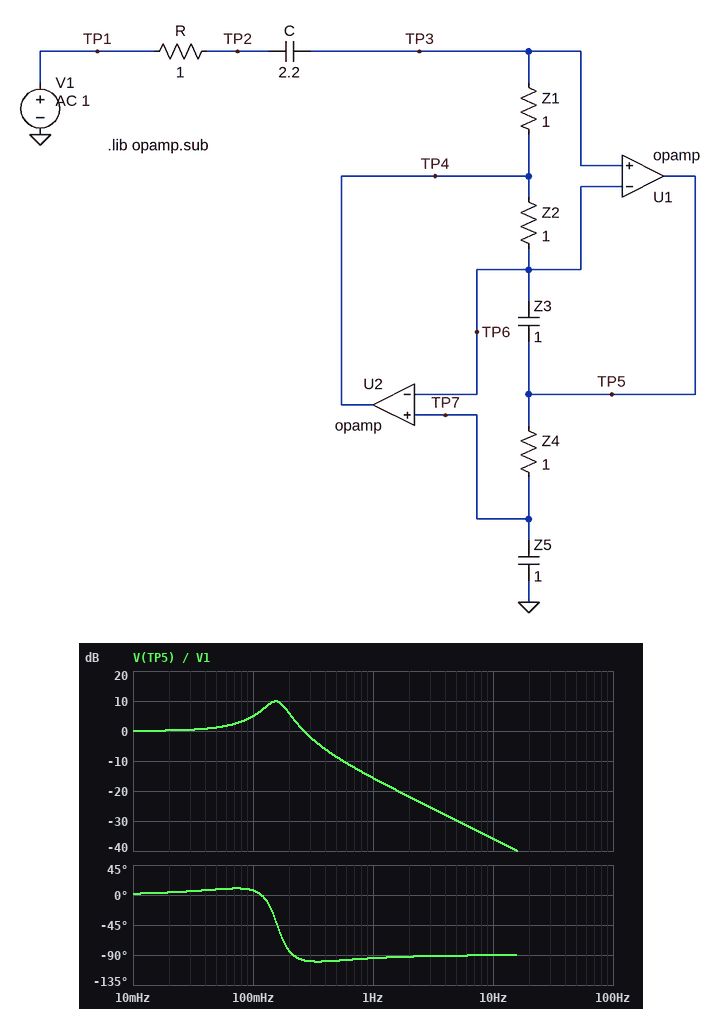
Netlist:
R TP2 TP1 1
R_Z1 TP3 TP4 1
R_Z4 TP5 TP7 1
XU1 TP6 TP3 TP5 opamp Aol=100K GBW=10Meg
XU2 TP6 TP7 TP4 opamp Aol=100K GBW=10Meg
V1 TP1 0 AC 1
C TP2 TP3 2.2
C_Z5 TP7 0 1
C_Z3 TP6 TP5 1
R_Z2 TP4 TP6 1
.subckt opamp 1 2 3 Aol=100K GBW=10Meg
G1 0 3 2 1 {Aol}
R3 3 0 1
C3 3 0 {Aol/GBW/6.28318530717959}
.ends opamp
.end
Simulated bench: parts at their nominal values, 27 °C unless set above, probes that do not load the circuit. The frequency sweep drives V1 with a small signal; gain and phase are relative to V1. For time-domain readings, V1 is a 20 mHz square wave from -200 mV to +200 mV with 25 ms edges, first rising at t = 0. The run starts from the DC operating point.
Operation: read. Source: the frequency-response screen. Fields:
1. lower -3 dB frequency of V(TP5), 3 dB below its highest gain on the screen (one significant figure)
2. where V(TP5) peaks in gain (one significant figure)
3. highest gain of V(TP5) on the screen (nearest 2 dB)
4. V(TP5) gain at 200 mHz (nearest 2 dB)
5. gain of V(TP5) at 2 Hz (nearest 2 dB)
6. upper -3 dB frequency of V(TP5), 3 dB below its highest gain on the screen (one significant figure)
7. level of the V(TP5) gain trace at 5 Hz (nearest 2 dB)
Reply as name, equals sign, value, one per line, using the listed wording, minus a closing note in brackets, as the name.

lower -3 dB frequency of V(TP5), 3 dB below its highest gain on the screen = 100 mHz
where V(TP5) peaks in gain = 200 mHz
highest gain of V(TP5) on the screen = 10 dB
V(TP5) gain at 200 mHz = 6 dB
gain of V(TP5) at 2 Hz = -22 dB
upper -3 dB frequency of V(TP5), 3 dB below its highest gain on the screen = 200 mHz
level of the V(TP5) gain trace at 5 Hz = -30 dB
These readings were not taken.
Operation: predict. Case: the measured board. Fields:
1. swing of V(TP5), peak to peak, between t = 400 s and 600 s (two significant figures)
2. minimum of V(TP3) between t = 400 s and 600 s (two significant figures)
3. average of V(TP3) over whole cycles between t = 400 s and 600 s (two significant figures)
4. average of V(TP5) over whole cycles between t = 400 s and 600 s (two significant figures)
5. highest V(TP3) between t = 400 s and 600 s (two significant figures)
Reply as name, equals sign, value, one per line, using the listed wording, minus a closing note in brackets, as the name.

swing of V(TP5), peak to peak, between t = 400 s and 600 s = 990 mV
minimum of V(TP3) between t = 400 s and 600 s = -190 mV
average of V(TP3) over whole cycles between t = 400 s and 600 s = 200 mV
average of V(TP5) over whole cycles between t = 400 s and 600 s = 200 mV
highest V(TP3) between t = 400 s and 600 s = 590 mV
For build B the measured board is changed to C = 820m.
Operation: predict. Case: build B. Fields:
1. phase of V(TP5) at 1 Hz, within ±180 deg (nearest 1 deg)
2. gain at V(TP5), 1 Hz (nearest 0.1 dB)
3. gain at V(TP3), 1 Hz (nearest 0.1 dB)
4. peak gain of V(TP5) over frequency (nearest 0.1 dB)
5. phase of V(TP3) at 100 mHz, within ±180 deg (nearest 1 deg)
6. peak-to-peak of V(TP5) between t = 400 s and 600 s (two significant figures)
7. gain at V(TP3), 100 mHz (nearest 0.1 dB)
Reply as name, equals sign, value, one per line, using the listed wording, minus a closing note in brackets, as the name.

phase of V(TP5) at 1 Hz, within ±180 deg = -88 deg
gain at V(TP5), 1 Hz = -15.8 dB
gain at V(TP3), 1 Hz = -31.9 dB
peak gain of V(TP5) over frequency = 1.8 dB
phase of V(TP3) at 100 mHz, within ±180 deg = -52 deg
peak-to-peak of V(TP5) between t = 400 s and 600 s = 550 mV
gain at V(TP3), 100 mHz = 0.2 dB
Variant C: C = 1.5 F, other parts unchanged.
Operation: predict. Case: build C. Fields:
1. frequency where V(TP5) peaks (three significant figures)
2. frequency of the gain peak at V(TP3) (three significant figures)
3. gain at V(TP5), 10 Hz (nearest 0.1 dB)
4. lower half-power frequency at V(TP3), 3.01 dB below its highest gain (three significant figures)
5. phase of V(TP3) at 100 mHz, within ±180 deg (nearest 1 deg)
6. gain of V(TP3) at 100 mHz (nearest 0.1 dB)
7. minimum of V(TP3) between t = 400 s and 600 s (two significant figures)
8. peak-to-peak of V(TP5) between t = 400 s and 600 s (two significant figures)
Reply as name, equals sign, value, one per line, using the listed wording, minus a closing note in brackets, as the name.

frequency where V(TP5) peaks = 150 mHz
frequency of the gain peak at V(TP3) = 140 mHz
gain at V(TP5), 10 Hz = -36.0 dB
lower half-power frequency at V(TP3), 3.01 dB below its highest gain = 61.5 mHz
phase of V(TP3) at 100 mHz, within ±180 deg = -35 deg
gain of V(TP3) at 100 mHz = 2.7 dB
minimum of V(TP3) between t = 400 s and 600 s = -130 mV
peak-to-peak of V(TP5) between t = 400 s and 600 s = 830 mV
